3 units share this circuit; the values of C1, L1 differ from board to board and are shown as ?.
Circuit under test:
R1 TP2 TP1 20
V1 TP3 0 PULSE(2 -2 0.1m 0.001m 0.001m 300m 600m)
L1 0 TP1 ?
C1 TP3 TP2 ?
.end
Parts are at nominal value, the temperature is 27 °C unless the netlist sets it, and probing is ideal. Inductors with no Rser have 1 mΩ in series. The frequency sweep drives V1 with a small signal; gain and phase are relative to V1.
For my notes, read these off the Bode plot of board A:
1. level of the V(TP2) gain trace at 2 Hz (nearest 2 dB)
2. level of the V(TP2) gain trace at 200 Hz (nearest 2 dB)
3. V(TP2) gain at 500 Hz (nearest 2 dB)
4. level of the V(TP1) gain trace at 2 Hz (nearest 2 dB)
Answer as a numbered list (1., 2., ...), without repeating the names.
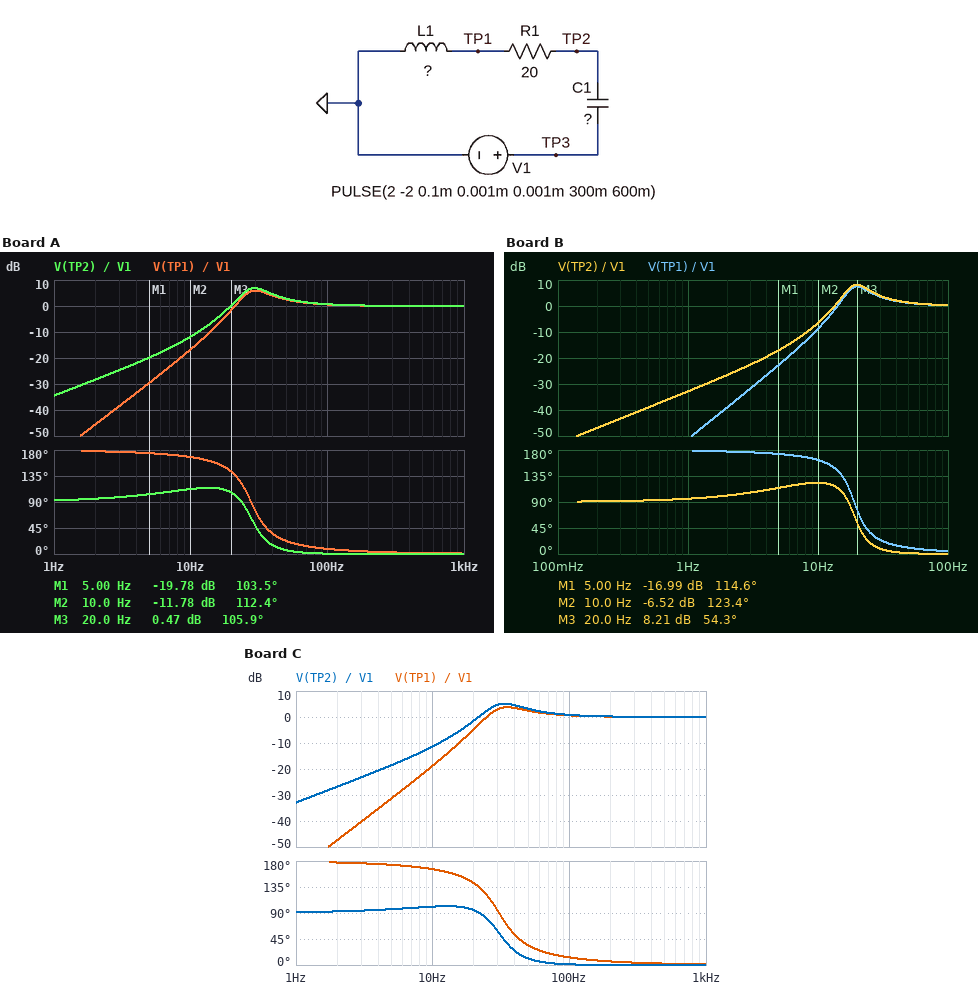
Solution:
1. -28 dB
2. 0 dB
3. 0 dB
4. -46 dB
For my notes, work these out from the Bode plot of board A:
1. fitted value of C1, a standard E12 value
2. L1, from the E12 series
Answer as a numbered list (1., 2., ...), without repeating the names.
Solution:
1. 150 µF
2. 220 mH
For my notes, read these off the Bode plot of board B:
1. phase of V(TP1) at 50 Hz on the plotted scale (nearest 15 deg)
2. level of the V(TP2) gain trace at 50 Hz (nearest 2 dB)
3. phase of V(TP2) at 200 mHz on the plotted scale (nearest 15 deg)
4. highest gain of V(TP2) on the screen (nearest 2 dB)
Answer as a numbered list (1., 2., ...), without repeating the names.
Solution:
1. 15 deg
2. 2 dB
3. 90 deg
4. 8 dB
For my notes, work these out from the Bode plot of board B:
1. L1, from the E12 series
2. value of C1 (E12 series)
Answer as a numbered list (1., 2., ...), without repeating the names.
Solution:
1. 390 mH
2. 180 µF
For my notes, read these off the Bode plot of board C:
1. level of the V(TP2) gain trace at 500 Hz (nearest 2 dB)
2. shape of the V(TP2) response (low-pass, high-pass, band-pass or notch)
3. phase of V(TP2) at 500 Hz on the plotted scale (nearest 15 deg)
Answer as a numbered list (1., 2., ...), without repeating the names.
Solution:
1. 0 dB
2. high-pass
3. 0 deg
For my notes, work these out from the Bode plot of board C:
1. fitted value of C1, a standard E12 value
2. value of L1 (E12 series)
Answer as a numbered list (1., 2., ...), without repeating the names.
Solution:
1. 180 µF
2. 150 mH
